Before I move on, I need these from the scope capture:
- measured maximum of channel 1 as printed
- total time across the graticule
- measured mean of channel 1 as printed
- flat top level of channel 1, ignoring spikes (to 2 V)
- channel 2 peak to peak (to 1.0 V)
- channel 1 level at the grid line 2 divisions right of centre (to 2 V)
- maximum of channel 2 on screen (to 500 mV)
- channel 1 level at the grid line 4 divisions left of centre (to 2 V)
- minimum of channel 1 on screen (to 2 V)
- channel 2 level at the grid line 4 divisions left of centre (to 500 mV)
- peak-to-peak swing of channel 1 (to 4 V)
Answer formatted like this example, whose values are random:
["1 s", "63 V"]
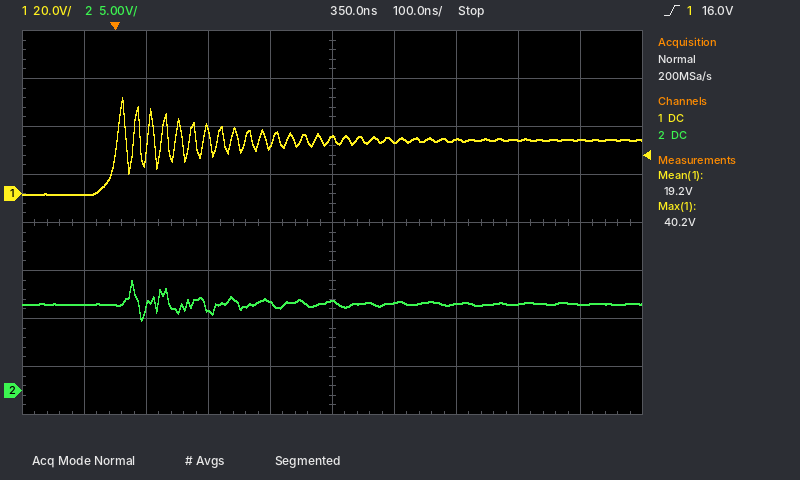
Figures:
["40.2 V", "1 µs", "19.2 V", "22 V", "4.0 V", "22 V", "11.5 V", "0 V", "0 V", "9.0 V", "40 V"]
